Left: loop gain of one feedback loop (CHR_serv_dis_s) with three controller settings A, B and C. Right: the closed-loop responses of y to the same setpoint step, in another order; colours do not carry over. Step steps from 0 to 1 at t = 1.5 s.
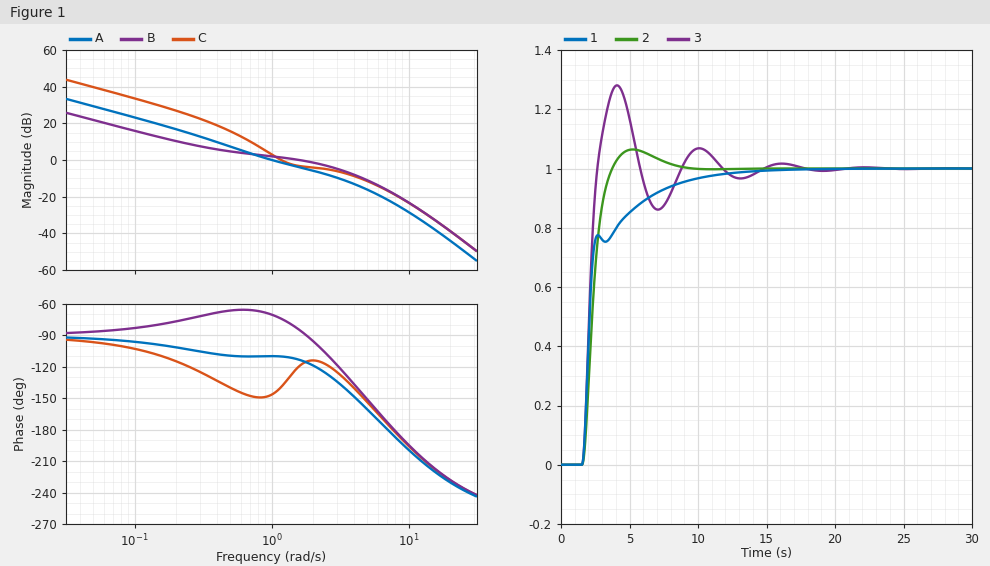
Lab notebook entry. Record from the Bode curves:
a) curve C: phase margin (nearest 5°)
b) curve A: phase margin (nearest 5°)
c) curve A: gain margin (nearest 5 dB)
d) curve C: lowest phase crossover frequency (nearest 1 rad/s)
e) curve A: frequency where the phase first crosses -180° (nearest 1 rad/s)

40°
70°
20 dB
8 rad/s
7 rad/s
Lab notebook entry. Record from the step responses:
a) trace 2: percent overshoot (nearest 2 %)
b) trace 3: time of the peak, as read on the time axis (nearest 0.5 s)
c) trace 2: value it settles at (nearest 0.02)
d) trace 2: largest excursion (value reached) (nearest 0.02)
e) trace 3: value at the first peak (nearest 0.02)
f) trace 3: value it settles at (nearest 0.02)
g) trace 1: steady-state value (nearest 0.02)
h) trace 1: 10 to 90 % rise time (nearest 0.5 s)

6 %
4.0 s
1.00
1.06
1.28
1.00
1.00
4.5 s
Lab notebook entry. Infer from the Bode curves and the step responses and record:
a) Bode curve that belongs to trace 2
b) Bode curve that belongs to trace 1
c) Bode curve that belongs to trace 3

A
B
C
